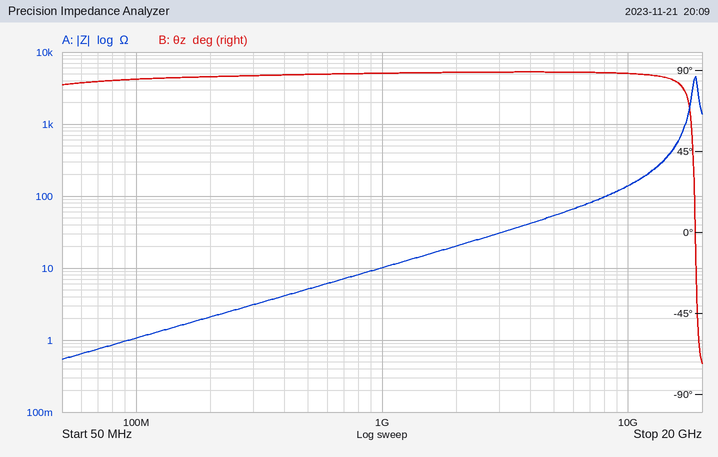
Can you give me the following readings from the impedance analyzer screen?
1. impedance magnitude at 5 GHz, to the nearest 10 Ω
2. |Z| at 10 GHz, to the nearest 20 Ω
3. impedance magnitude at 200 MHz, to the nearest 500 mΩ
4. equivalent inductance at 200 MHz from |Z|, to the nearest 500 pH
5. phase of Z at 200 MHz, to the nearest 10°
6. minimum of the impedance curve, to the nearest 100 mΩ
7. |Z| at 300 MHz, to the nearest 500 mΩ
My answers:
50 Ω
140 Ω
2.0 Ω
1.5 nH
90°
500 mΩ
3.0 Ω
